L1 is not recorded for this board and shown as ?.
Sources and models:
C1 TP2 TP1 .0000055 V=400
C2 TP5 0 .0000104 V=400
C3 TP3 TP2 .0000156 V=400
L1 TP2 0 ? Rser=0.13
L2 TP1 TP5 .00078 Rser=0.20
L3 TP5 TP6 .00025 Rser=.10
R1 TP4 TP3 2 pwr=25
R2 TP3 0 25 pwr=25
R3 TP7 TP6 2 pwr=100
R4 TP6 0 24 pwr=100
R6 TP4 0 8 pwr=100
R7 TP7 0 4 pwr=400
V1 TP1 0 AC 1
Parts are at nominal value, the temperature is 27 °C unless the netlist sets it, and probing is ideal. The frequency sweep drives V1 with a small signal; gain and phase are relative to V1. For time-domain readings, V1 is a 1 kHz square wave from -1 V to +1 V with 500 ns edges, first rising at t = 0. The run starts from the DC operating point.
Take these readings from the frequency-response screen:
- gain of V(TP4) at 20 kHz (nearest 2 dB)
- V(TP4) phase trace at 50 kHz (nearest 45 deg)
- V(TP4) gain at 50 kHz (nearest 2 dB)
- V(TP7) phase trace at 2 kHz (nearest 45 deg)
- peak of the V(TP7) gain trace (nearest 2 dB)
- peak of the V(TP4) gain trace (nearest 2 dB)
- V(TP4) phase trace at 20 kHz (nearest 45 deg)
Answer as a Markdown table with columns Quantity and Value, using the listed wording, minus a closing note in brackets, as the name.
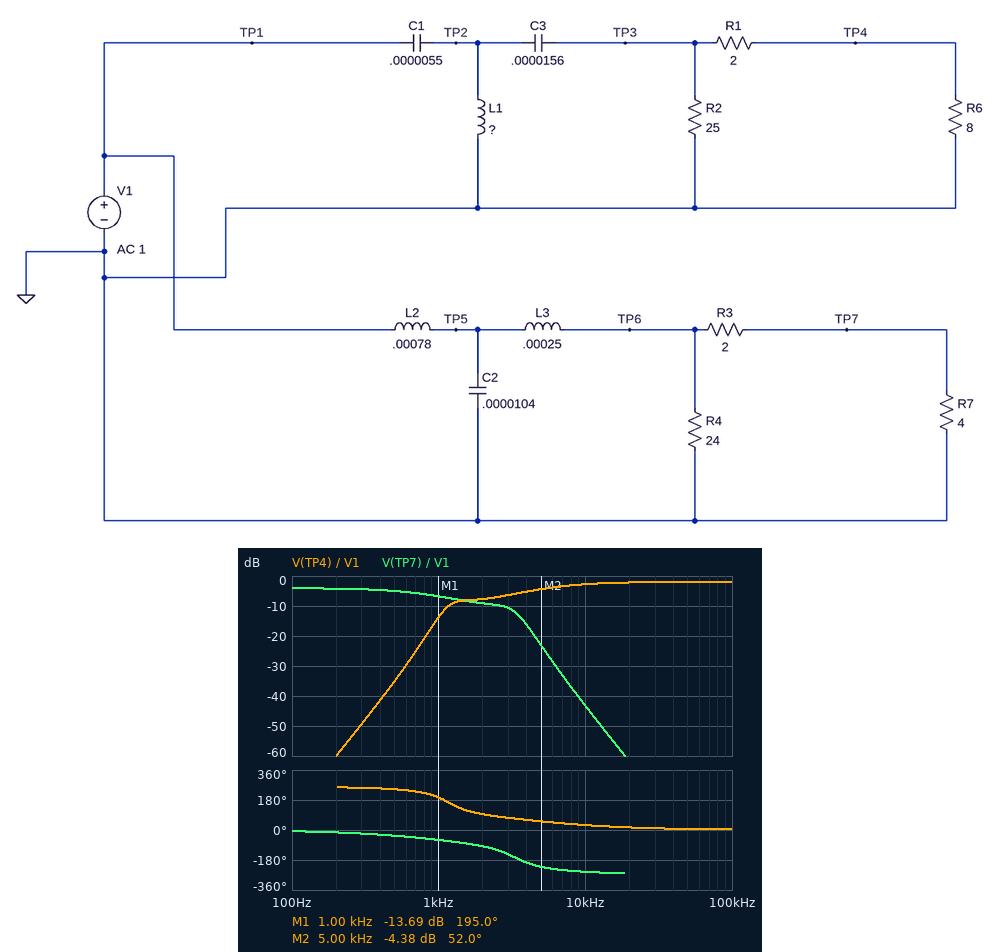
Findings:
| Quantity | Value |
|---|---|
| gain of V(TP4) at 20 kHz | -2 dB |
| V(TP4) phase trace at 50 kHz | 0 deg |
| V(TP4) gain at 50 kHz | -2 dB |
| V(TP7) phase trace at 2 kHz | -90 deg |
| peak of the V(TP7) gain trace | -4 dB |
| peak of the V(TP4) gain trace | -2 dB |
| V(TP4) phase trace at 20 kHz | 0 deg |
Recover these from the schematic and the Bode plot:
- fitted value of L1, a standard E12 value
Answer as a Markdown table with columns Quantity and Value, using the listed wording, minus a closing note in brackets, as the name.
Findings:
| Quantity | Value |
|---|---|
| fitted value of L1, a standard E12 value | 1 mH |
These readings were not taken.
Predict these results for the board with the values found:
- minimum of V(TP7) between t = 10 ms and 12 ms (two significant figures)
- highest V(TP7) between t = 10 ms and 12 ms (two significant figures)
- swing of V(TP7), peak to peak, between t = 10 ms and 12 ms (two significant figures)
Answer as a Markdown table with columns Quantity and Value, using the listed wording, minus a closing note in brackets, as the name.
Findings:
| Quantity | Value |
|---|---|
| minimum of V(TP7) between t = 10 ms and 12 ms | -560 mV |
| highest V(TP7) between t = 10 ms and 12 ms | 560 mV |
| swing of V(TP7), peak to peak, between t = 10 ms and 12 ms | 1.1 V |
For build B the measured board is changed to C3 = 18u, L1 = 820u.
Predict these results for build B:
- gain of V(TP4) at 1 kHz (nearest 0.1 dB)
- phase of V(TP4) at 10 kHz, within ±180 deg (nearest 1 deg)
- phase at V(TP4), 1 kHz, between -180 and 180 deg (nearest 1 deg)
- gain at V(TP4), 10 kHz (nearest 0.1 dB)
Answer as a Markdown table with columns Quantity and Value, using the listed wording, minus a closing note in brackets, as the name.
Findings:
| Quantity | Value |
|---|---|
| gain of V(TP4) at 1 kHz | -16.0 dB |
| phase of V(TP4) at 10 kHz, within ±180 deg | 29 deg |
| phase at V(TP4), 1 kHz, between -180 and 180 deg | -162 deg |
| gain at V(TP4), 10 kHz | -2.6 dB |
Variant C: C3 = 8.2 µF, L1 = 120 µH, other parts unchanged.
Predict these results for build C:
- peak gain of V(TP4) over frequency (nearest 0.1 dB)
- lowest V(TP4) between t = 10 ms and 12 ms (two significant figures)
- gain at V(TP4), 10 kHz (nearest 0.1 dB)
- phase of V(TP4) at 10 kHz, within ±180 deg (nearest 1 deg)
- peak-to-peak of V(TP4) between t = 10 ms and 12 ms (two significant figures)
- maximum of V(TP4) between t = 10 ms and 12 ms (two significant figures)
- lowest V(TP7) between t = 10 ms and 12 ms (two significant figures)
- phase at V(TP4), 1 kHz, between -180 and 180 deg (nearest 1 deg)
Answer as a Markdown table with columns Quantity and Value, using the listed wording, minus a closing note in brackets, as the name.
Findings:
| Quantity | Value |
|---|---|
| peak gain of V(TP4) over frequency | 1.4 dB |
| lowest V(TP4) between t = 10 ms and 12 ms | -1.6 V |
| gain at V(TP4), 10 kHz | -0.5 dB |
| phase of V(TP4) at 10 kHz, within ±180 deg | 43 deg |
| peak-to-peak of V(TP4) between t = 10 ms and 12 ms | 3.2 V |
| maximum of V(TP4) between t = 10 ms and 12 ms | 1.6 V |
| lowest V(TP7) between t = 10 ms and 12 ms | -560 mV |
| phase at V(TP4), 1 kHz, between -180 and 180 deg | -121 deg |
